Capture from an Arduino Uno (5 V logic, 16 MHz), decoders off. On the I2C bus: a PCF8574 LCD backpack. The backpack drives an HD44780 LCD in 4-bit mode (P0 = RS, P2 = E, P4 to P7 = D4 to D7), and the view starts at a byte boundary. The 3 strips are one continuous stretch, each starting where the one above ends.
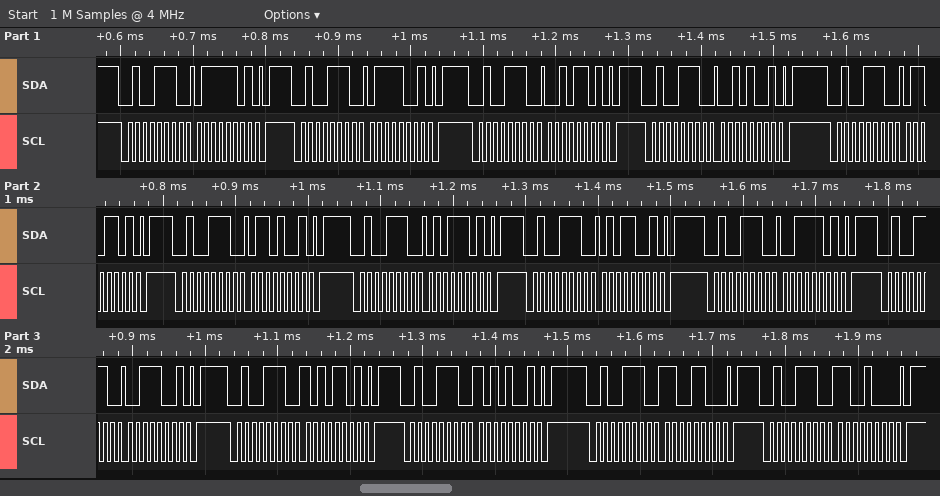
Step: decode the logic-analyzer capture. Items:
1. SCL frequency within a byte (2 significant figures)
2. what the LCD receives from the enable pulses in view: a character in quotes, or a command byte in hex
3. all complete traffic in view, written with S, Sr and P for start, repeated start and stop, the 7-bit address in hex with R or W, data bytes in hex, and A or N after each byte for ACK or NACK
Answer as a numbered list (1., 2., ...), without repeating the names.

1. 100 kHz
2. 'r' 'e' ':'
3. S 27W A 7D A P S 27W A 79 A P S 27W A 2D A P S 27W A 29 A P S 27W A 6D A P S 27W A 69 A P S 27W A 5D A P S 27W A 59 A P S 27W A 3D A P S 27W A 39 A P S 27W A AD A P S 27W A A9 A P S 27W A CC A P S 27W A C8 A P
